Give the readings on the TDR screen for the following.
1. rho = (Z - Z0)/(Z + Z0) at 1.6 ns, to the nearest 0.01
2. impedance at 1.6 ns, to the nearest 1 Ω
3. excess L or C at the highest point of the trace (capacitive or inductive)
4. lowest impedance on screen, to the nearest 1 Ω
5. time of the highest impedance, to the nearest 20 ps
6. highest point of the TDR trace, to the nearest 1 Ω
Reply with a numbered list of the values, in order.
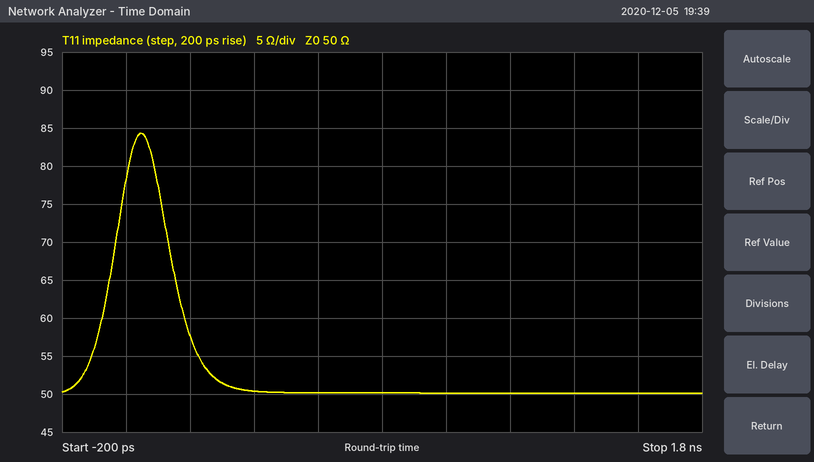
1. 0.00
2. 50 Ω
3. inductive
4. 50 Ω
5. 40 ps
6. 84 Ω
